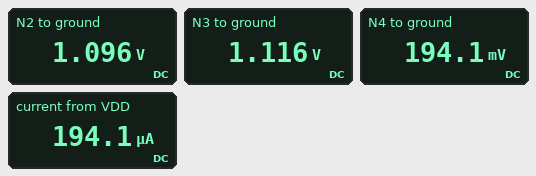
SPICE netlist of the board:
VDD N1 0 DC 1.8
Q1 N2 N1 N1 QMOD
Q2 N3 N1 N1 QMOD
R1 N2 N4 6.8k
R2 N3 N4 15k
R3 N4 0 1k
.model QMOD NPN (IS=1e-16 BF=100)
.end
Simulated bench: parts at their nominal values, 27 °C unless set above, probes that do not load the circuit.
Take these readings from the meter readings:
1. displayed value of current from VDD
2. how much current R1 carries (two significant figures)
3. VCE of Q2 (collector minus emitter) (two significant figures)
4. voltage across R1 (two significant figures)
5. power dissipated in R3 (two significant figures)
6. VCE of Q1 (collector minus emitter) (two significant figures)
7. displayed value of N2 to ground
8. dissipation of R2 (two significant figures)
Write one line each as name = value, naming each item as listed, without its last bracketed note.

displayed value of current from VDD = 194.1 µA
how much current R1 carries = 130 µA
VCE of Q2 (collector minus emitter) = -680 mV
voltage across R1 = 900 mV
power dissipated in R3 = 38 µW
VCE of Q1 (collector minus emitter) = -700 mV
displayed value of N2 to ground = 1.096 V
dissipation of R2 = 57 µW
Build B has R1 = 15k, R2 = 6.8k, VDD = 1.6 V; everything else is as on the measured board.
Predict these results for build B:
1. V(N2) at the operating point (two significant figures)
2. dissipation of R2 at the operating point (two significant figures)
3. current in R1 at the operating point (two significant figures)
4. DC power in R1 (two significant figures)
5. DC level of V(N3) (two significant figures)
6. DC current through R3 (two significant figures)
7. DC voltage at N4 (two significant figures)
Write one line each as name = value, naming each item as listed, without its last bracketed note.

V(N2) at the operating point = 920 mV
dissipation of R2 at the operating point = 81 µW
current in R1 at the operating point = 51 µA
DC power in R1 = 39 µW
DC level of V(N3) = 900 mV
DC current through R3 = 160 µA
DC voltage at N4 = 160 mV
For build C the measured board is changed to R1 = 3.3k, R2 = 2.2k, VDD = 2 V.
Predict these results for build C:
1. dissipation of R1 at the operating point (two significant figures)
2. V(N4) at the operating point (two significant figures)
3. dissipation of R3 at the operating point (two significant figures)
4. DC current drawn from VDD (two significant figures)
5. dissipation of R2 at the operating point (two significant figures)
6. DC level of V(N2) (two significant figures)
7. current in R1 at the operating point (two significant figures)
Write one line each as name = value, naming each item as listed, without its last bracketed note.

dissipation of R1 at the operating point = 160 µW
V(N4) at the operating point = 550 mV
dissipation of R3 at the operating point = 300 µW
DC current drawn from VDD = 550 µA
dissipation of R2 at the operating point = 240 µW
DC level of V(N2) = 1.3 V
current in R1 at the operating point = 220 µA
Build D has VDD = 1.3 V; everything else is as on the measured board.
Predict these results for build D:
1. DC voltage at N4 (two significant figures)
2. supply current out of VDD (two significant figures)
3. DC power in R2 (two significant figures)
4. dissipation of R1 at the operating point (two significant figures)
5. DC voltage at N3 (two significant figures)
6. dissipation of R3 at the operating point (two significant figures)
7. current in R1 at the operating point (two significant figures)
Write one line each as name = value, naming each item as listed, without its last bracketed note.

DC voltage at N4 = 110 mV
supply current out of VDD = 110 µA
DC power in R2 = 18 µW
dissipation of R1 at the operating point = 37 µW
DC voltage at N3 = 630 mV
dissipation of R3 at the operating point = 12 µW
current in R1 at the operating point = 74 µA
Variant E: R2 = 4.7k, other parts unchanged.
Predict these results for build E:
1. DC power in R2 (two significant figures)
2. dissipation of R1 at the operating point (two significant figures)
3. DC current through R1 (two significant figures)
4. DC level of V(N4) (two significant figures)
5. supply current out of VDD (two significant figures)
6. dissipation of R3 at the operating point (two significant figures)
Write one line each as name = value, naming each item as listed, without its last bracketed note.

DC power in R2 = 140 µW
dissipation of R1 at the operating point = 96 µW
DC current through R1 = 120 µA
DC level of V(N4) = 290 mV
supply current out of VDD = 290 µA
dissipation of R3 at the operating point = 84 µW
